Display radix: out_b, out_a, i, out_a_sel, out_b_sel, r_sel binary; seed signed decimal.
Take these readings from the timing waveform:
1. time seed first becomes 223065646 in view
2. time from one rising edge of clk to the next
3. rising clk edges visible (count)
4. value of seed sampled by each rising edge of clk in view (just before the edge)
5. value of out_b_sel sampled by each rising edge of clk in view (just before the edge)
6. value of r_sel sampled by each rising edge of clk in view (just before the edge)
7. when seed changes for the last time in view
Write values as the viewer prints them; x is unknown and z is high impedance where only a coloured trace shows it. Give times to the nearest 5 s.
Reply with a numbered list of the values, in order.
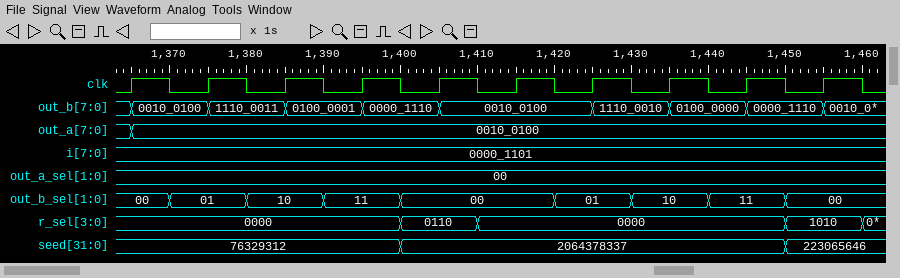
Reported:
1. 1450 s
2. 10 s
3. 10
4. 76329312, 76329312, 76329312, 76329312, 2064378337, 2064378337, 2064378337, 2064378337, 2064378337, 223065646
5. 00, 01, 10, 11, 00, 00, 01, 10, 11, 00
6. 0000, 0000, 0000, 0000, 0110, 0000, 0000, 0000, 0000, 1010
7. 1450 s
